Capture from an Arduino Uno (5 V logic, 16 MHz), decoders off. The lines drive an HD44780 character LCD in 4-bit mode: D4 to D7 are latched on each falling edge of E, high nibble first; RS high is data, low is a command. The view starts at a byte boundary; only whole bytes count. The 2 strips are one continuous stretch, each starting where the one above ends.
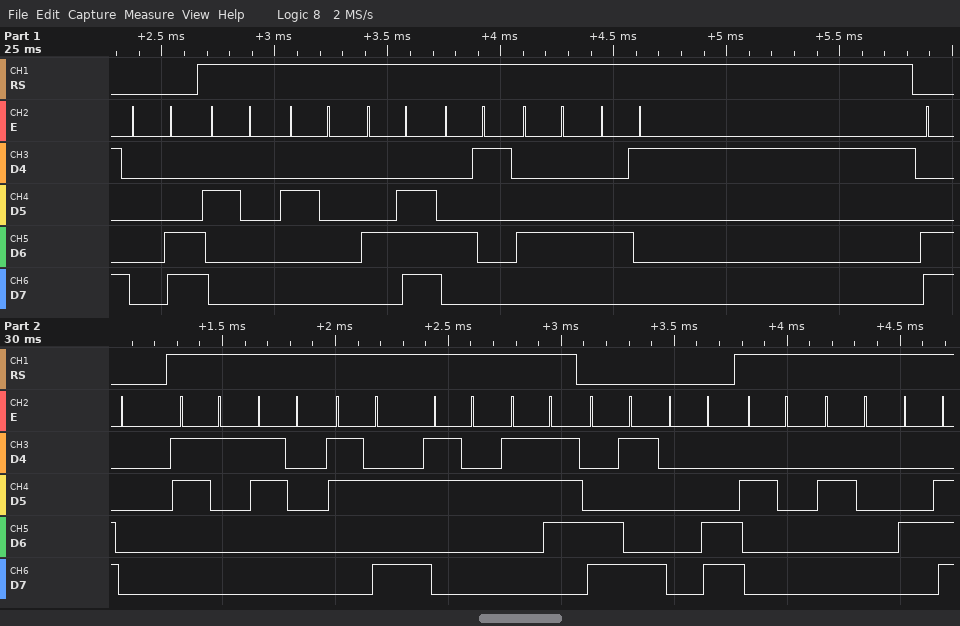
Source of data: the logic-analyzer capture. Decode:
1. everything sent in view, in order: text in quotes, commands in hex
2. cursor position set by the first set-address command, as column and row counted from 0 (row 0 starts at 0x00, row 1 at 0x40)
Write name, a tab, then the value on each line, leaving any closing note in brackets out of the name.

everything sent in view, in order: text in quotes, commands in hex	0x0C "  NADA" 0xC0 "10:27" 0xC9 0x0C "  N"
cursor position set by the first set-address command, as column and row counted from 0	column 0, row 1
